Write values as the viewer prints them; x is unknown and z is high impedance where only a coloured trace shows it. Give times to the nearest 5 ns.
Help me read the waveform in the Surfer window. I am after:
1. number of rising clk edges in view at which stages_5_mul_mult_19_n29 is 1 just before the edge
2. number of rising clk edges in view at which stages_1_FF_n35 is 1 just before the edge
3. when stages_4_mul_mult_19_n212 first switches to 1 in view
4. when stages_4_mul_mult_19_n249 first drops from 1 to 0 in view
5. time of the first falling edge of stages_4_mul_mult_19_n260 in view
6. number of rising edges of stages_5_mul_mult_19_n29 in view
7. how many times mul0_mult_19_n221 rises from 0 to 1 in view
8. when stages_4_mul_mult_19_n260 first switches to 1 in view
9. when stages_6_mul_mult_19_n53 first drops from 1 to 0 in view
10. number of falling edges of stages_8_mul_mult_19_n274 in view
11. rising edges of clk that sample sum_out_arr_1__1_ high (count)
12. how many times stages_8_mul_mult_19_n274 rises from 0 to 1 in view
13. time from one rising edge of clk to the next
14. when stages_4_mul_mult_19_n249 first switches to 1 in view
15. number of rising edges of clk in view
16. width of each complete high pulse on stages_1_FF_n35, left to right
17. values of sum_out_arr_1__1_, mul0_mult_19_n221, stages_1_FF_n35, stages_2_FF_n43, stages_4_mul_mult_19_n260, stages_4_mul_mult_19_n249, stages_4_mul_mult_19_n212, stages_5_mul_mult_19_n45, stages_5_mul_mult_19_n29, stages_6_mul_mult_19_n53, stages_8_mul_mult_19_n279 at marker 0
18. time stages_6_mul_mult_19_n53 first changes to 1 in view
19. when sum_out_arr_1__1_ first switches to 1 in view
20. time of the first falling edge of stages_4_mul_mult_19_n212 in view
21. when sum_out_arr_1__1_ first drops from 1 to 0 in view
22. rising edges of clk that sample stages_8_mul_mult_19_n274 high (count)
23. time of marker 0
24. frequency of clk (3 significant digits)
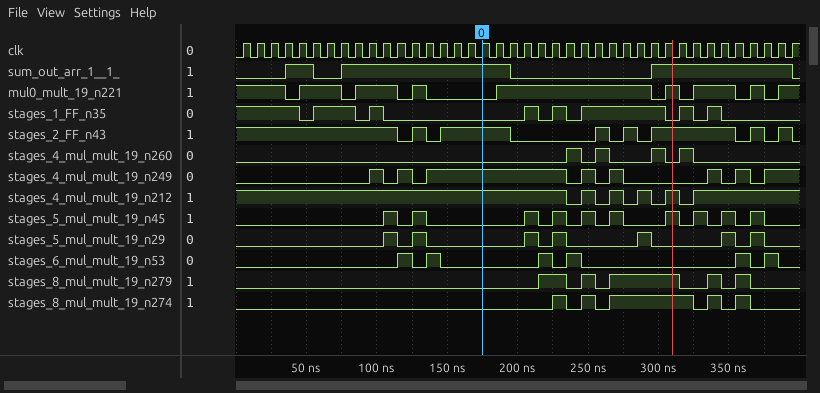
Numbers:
7
19
245 ns
105 ns
245 ns
7
8
235 ns
125 ns
5
24
5
10 ns
95 ns
40
30 ns, 10 ns, 10 ns, 10 ns, 60 ns, 10 ns, 10 ns
sum_out_arr_1__1_=1, mul0_mult_19_n221=0, stages_1_FF_n35=0, stages_2_FF_n43=1, stages_4_mul_mult_19_n260=0, stages_4_mul_mult_19_n249=1, stages_4_mul_mult_19_n212=1, stages_5_mul_mult_19_n45=0, stages_5_mul_mult_19_n29=0, stages_6_mul_mult_19_n53=0, stages_8_mul_mult_19_n279=0
115 ns
35 ns
235 ns
55 ns
10
175 ns
100 MHz
